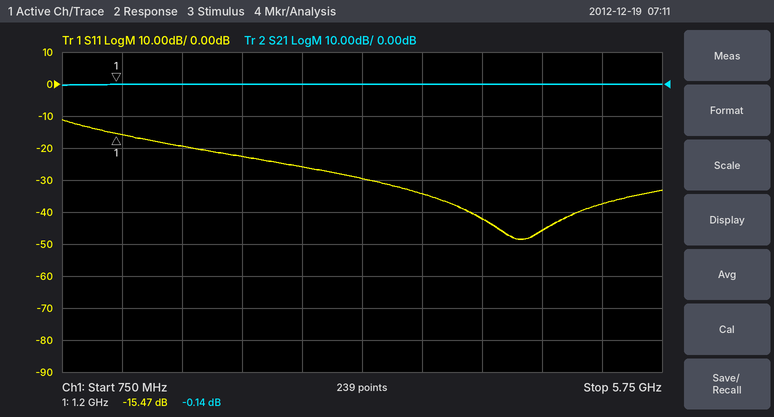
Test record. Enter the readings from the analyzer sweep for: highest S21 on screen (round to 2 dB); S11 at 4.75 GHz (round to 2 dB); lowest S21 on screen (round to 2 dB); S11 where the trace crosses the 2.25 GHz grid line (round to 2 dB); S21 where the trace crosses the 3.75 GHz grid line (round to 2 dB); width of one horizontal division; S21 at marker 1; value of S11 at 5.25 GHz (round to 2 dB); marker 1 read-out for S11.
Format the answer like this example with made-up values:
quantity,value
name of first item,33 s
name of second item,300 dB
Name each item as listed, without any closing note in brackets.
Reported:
quantity,value
highest S21 on screen,0 dB
S11 at 4.75 GHz,-46 dB
lowest S21 on screen,0 dB
S11 where the trace crosses the 2.25 GHz grid line,-22 dB
S21 where the trace crosses the 3.75 GHz grid line,0 dB
width of one horizontal division,500 MHz
S21 at marker 1,-0.14 dB
value of S11 at 5.25 GHz,-38 dB
marker 1 read-out for S11,-15.47 dB
